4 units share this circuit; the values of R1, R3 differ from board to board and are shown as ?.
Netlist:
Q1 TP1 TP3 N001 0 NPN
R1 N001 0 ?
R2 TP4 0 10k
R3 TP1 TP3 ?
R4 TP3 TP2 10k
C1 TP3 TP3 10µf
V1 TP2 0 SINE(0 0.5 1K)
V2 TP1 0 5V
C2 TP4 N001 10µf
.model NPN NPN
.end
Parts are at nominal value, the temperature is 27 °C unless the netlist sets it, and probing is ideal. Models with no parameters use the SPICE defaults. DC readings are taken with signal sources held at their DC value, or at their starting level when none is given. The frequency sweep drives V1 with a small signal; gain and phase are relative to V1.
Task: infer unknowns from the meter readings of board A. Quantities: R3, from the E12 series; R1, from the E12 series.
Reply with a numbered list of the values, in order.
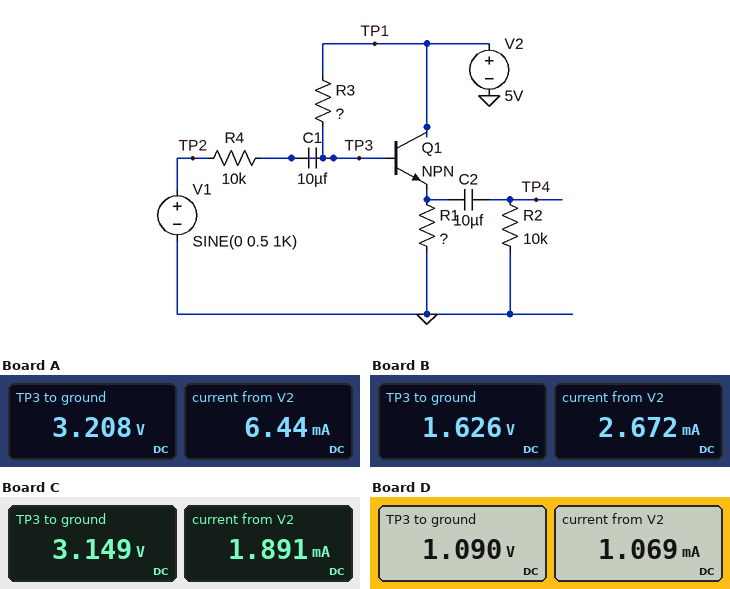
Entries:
1. 4.7 kΩ
2. 390 Ω
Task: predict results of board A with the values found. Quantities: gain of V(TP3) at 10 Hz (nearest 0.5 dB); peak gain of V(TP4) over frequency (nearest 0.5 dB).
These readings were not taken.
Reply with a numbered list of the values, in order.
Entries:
1. -10.5 dB
2. -10.5 dB
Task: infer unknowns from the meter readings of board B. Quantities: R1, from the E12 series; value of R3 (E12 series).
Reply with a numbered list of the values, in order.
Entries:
1. 330 Ω
2. 18 kΩ
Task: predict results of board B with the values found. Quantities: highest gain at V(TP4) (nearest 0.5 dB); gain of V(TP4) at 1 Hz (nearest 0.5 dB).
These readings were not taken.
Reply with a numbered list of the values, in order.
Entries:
1. -5.5 dB
2. -11.0 dB
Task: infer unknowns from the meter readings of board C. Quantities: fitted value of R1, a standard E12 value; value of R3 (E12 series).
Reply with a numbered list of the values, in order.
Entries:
1. 1.5 kΩ
2. 5.6 kΩ
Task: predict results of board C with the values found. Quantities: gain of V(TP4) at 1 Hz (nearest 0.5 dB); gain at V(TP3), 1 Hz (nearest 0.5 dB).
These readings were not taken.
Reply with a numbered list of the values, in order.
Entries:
1. -14.5 dB
2. -9.0 dB
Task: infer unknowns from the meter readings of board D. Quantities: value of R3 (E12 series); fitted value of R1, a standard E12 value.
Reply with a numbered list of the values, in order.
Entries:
1. 33 kΩ
2. 330 Ω
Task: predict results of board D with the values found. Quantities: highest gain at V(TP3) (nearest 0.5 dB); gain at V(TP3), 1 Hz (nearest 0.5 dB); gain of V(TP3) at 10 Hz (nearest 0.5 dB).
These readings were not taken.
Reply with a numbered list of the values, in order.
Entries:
1. -4.0 dB
2. -4.0 dB
3. -4.0 dB
